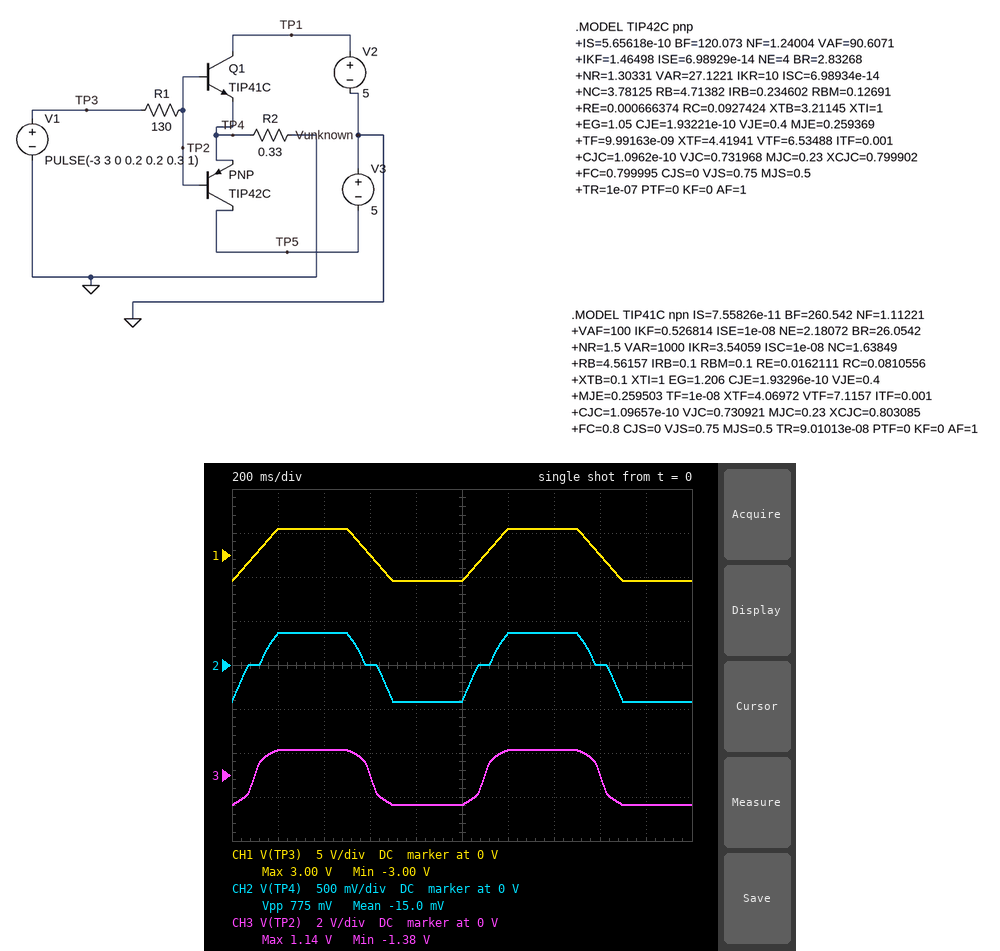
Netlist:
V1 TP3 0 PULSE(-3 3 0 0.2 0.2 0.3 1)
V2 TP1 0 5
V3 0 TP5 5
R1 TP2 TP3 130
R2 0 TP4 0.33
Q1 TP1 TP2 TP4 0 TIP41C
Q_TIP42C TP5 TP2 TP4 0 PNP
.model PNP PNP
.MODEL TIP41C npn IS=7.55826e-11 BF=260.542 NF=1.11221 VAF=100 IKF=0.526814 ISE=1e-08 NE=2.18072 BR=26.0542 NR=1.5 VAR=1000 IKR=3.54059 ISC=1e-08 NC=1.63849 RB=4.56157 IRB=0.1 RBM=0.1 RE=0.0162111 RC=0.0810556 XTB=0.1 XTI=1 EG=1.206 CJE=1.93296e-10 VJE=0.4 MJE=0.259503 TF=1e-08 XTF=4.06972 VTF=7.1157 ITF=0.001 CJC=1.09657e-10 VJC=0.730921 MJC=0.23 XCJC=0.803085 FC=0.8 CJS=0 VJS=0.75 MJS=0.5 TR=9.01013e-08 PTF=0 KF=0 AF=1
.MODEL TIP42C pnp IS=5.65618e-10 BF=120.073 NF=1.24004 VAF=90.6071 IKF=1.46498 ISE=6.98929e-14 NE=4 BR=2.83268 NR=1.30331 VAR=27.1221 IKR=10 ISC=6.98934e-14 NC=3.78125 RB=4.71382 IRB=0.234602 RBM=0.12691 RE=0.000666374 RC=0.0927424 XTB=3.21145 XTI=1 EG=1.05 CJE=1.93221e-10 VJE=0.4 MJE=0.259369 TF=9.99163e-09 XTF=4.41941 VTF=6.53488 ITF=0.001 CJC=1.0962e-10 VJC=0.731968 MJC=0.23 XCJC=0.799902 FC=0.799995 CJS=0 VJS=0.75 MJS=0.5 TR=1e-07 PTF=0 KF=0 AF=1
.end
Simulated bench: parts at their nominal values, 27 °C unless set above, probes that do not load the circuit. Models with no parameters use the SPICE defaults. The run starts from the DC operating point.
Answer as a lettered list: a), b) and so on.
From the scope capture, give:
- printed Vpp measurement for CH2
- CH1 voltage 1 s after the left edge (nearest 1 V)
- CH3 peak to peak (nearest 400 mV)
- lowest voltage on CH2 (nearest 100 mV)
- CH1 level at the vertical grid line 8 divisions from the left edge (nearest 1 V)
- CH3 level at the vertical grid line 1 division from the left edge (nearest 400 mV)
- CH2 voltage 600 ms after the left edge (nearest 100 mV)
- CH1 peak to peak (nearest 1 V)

a) 775 mV
b) -3 V
c) 2.4 V
d) -400 mV
e) 0 V
f) 1.2 V
g) 0 V
h) 6 V
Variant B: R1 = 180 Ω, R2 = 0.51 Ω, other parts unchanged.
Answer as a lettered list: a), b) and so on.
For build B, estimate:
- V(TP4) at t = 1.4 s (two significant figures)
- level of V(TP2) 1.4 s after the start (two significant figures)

a) 440 mV
b) 1.2 V
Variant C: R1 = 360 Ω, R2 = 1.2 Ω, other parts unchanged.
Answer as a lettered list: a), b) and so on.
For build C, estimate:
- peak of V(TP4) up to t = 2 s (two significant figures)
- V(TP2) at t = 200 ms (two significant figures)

a) 590 mV
b) 1.3 V
